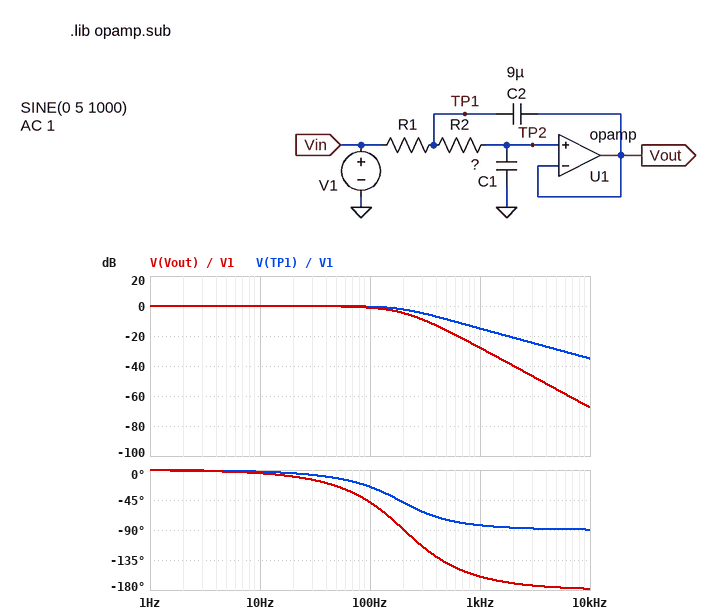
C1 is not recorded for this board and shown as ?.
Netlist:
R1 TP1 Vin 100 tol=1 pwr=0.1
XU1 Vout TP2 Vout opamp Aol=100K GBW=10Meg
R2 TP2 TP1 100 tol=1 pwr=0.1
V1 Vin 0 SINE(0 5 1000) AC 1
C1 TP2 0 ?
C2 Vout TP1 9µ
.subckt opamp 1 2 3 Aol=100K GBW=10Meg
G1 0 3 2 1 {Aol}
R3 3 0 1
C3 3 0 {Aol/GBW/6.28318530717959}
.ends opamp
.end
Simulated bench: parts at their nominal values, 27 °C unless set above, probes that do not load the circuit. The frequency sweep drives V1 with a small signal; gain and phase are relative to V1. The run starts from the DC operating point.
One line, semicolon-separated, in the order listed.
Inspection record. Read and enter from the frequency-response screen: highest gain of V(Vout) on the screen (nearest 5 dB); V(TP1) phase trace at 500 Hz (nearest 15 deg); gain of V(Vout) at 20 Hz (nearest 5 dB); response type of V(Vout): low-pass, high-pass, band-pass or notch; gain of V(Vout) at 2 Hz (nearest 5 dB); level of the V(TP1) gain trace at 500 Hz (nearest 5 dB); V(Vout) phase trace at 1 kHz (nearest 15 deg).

0 dB; -75 deg; 0 dB; low-pass; 0 dB; -10 dB; -165 deg
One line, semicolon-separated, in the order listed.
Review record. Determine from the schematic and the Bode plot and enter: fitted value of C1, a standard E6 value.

6.8 µF
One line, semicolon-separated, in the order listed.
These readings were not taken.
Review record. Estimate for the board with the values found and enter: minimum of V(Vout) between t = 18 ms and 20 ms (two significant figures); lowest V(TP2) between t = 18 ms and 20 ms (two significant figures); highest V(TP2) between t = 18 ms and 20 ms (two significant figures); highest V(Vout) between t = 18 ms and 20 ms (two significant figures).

-200 mV; -200 mV; 200 mV; 200 mV
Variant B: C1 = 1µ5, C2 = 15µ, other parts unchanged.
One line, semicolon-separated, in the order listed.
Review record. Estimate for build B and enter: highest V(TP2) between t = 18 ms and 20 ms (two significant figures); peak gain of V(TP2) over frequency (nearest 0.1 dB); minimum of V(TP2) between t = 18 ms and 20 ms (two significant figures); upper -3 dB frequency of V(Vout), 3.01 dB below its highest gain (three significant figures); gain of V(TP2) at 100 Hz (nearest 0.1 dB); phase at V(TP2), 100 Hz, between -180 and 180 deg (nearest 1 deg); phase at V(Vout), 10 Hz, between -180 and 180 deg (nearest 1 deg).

620 mV; 4.4 dB; -620 mV; 397 Hz; 0.6 dB; -12 deg; -1 deg
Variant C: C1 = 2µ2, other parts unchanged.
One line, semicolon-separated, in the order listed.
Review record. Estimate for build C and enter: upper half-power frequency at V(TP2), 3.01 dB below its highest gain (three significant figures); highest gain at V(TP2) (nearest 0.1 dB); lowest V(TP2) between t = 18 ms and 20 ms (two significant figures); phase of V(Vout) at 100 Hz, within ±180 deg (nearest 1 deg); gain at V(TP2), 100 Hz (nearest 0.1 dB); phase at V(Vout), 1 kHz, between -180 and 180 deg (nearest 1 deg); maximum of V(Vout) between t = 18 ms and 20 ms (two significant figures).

419 Hz; 1.3 dB; -680 mV; -17 deg; 0.3 dB; -158 deg; 680 mV
